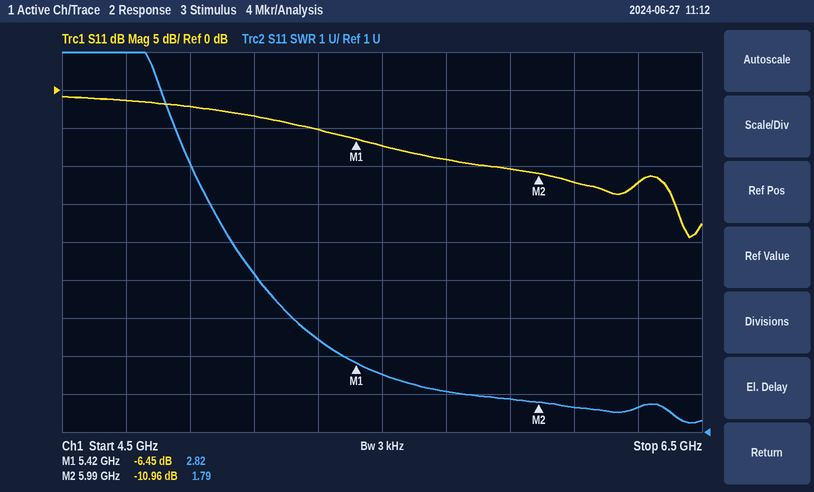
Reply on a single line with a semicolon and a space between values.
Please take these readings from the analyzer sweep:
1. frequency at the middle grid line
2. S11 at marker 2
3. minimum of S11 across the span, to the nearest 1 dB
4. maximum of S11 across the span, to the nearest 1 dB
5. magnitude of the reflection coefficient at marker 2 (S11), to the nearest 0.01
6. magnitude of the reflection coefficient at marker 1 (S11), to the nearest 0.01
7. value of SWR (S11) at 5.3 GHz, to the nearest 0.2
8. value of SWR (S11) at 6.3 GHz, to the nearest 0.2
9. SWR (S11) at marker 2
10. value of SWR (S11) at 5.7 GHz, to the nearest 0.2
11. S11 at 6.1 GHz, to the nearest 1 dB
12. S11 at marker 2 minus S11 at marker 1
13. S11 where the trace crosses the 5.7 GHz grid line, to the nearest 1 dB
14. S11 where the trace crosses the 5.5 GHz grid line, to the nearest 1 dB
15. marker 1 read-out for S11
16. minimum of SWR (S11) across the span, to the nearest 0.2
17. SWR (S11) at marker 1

5.5 GHz; -10.96 dB; -19 dB; -1 dB; 0.28; 0.48; 3.4; 1.6; 1.79; 2.0; -12 dB; -4.51 dB; -9 dB; -7 dB; -6.45 dB; 1.2; 2.82
